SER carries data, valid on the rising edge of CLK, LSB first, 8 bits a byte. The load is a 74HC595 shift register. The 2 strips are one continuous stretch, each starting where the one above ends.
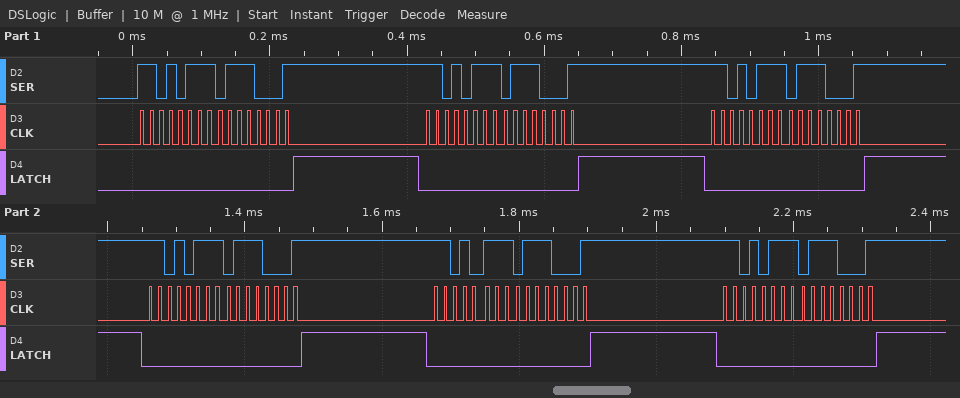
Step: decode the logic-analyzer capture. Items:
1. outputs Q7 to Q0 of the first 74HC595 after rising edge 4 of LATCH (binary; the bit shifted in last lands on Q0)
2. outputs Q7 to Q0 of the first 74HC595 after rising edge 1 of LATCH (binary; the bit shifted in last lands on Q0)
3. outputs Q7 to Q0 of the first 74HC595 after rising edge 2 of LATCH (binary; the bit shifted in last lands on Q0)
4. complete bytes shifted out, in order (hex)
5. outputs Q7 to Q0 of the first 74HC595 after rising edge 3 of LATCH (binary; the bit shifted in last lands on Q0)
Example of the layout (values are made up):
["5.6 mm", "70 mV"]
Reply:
["01110001", "01110001", "01110001", "EB 8E EB 8E EB 8E EB 8E EB 8E EB 8E", "01110001"]
